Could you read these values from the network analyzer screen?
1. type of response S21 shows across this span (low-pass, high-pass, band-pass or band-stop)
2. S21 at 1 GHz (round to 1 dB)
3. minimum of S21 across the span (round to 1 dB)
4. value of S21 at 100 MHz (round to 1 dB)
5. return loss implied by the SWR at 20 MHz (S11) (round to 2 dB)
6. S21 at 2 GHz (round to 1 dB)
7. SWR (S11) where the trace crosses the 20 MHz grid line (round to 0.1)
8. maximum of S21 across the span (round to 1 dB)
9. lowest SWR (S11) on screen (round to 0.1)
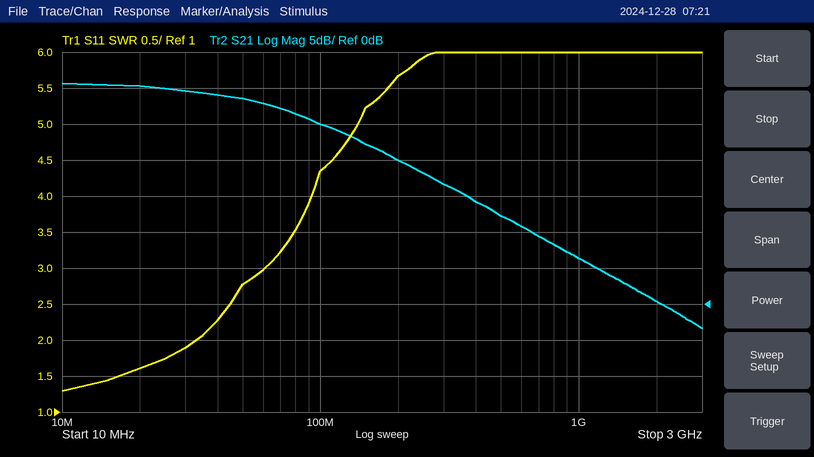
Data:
low-pass
6 dB
-3 dB
25 dB
12 dB
0 dB
1.6
31 dB
1.3
